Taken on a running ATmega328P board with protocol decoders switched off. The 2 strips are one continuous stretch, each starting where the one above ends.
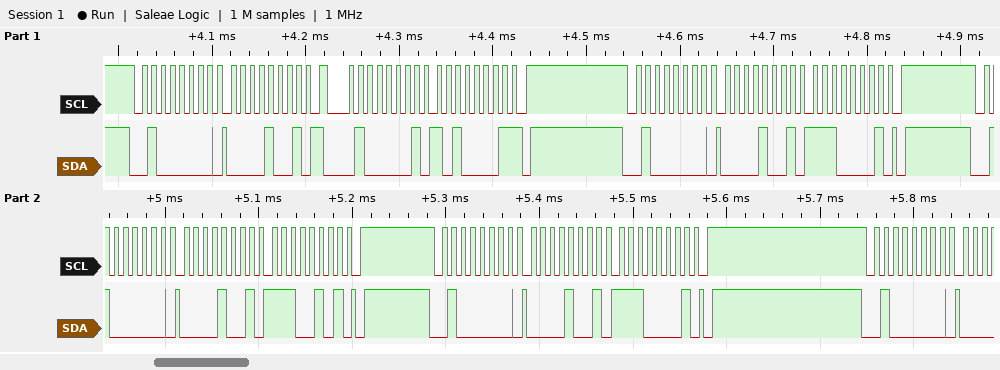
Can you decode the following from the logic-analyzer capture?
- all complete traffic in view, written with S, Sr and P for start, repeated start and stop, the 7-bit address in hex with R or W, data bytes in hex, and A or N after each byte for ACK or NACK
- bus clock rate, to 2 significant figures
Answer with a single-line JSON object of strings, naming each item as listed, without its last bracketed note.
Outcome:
{"all complete traffic in view, written with S, Sr and P for start, repeated start and stop, the 7-bit address in hex with R or W, data bytes in hex, and A or N after each byte for ACK or NACK": "S 20W A 09 A Sr 20R A A1 N P S 20W A 09 A E1 A P S 20W A 09 A E5 A P S 20W A 09 A E1 A P S 20W A", "bus clock rate, to 2 significant figures": "100 kHz"}
